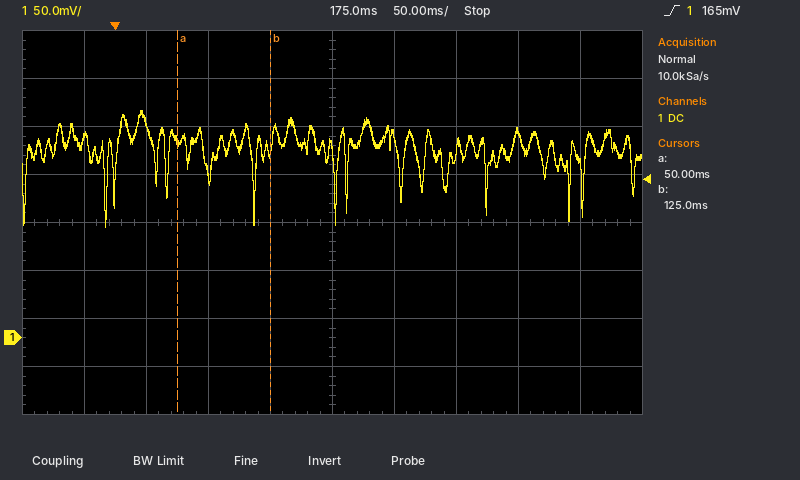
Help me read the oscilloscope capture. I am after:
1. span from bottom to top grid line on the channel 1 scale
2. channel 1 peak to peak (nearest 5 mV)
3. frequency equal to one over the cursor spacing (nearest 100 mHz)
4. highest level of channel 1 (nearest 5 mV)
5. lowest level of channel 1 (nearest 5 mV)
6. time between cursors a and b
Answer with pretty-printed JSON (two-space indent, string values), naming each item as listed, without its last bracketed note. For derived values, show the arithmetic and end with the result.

{
  "span from bottom to top grid line on the channel 1 scale": "400 mV",
  "channel 1 peak to peak": "235 mV − (115 mV) = 120 mV",
  "frequency equal to one over the cursor spacing": "1 / 75 ms ≈ 13.3 Hz",
  "highest level of channel 1": "235 mV",
  "lowest level of channel 1": "115 mV",
  "time between cursors a and b": "125 ms − (50 ms) = 75 ms"
}
